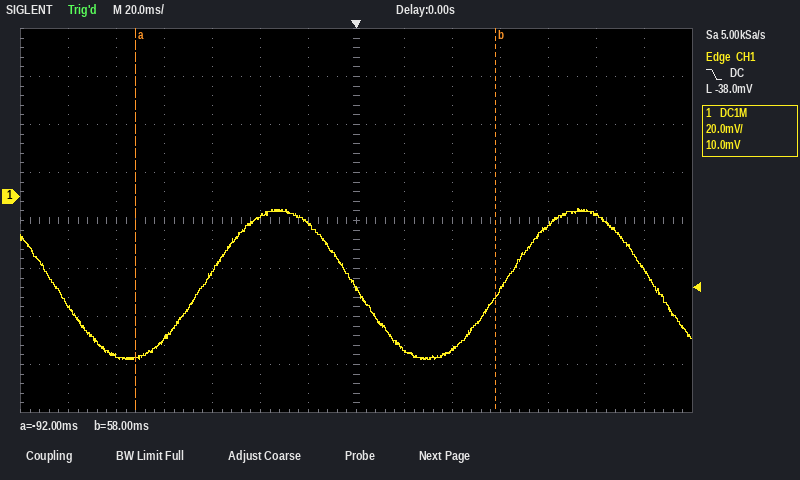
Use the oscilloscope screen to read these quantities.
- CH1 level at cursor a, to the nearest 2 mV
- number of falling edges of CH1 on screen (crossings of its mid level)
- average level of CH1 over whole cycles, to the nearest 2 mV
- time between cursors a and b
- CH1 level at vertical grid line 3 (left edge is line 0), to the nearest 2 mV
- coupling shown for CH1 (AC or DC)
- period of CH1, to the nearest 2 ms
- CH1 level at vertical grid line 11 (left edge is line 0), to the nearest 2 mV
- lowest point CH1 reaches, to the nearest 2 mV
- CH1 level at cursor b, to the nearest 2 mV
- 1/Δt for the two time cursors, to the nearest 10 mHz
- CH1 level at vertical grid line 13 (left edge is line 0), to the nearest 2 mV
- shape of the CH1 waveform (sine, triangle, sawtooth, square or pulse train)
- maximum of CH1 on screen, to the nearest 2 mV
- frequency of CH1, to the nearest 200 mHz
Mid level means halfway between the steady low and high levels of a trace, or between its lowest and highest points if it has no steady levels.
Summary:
-68 mV
3
-36 mV
150 ms
-60 mV
DC
124 ms
-12 mV
-68 mV
-42 mV
6.67 Hz
-30 mV
sine
-4 mV
8.0 Hz
